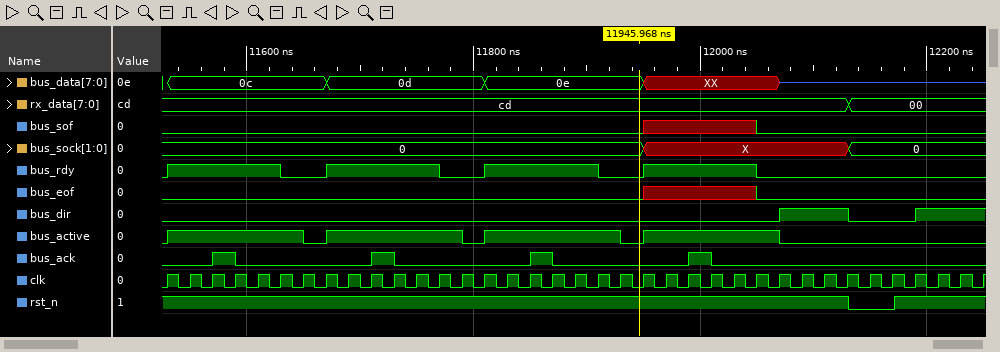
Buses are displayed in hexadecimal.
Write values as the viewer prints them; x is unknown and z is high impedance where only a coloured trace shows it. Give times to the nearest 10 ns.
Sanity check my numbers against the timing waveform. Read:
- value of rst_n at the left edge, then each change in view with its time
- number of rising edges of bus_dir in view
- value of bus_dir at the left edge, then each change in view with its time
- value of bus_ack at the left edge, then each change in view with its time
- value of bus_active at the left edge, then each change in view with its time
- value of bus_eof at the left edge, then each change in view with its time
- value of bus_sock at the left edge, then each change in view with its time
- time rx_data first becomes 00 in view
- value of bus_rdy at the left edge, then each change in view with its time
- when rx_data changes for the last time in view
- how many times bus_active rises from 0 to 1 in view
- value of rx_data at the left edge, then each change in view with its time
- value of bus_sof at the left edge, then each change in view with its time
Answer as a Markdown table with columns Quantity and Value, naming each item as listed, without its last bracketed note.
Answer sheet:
| Quantity | Value |
|---|---|
| value of rst_n at the left edge, then each change in view with its time | 1, 0 at 12130 ns, 1 at 12170 ns |
| number of rising edges of bus_dir in view | 2 |
| value of bus_dir at the left edge, then each change in view with its time | 0, 1 at 12070 ns, 0 at 12130 ns, 1 at 12190 ns |
| value of bus_ack at the left edge, then each change in view with its time | 0, 1 at 11570 ns, 0 at 11590 ns, 1 at 11710 ns, 0 at 11730 ns, 1 at 11850 ns, 0 at 11870 ns, 1 at 11990 ns, 0 at 12010 ns |
| value of bus_active at the left edge, then each change in view with its time | 0, 1 at 11530 ns, 0 at 11650 ns, 1 at 11670 ns, 0 at 11790 ns, 1 at 11810 ns, 0 at 11930 ns, 1 at 11950 ns, 0 at 12070 ns |
| value of bus_eof at the left edge, then each change in view with its time | 0, x at 11950 ns, 0 at 12050 ns |
| value of bus_sock at the left edge, then each change in view with its time | 0, X at 11950 ns, 0 at 12130 ns |
| time rx_data first becomes 00 in view | 12130 ns |
| value of bus_rdy at the left edge, then each change in view with its time | 0, 1 at 11530 ns, 0 at 11630 ns, 1 at 11670 ns, 0 at 11770 ns, 1 at 11810 ns, 0 at 11910 ns, 1 at 11950 ns, 0 at 12050 ns |
| when rx_data changes for the last time in view | 12130 ns |
| how many times bus_active rises from 0 to 1 in view | 4 |
| value of rx_data at the left edge, then each change in view with its time | cd, 00 at 12130 ns |
| value of bus_sof at the left edge, then each change in view with its time | 0, x at 11950 ns, 0 at 12050 ns |
